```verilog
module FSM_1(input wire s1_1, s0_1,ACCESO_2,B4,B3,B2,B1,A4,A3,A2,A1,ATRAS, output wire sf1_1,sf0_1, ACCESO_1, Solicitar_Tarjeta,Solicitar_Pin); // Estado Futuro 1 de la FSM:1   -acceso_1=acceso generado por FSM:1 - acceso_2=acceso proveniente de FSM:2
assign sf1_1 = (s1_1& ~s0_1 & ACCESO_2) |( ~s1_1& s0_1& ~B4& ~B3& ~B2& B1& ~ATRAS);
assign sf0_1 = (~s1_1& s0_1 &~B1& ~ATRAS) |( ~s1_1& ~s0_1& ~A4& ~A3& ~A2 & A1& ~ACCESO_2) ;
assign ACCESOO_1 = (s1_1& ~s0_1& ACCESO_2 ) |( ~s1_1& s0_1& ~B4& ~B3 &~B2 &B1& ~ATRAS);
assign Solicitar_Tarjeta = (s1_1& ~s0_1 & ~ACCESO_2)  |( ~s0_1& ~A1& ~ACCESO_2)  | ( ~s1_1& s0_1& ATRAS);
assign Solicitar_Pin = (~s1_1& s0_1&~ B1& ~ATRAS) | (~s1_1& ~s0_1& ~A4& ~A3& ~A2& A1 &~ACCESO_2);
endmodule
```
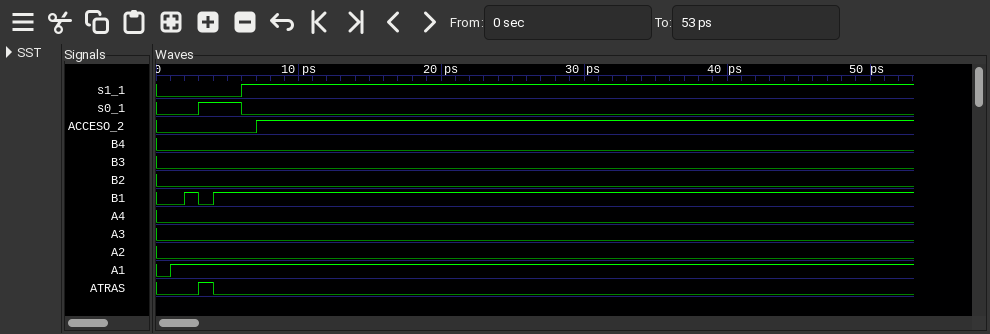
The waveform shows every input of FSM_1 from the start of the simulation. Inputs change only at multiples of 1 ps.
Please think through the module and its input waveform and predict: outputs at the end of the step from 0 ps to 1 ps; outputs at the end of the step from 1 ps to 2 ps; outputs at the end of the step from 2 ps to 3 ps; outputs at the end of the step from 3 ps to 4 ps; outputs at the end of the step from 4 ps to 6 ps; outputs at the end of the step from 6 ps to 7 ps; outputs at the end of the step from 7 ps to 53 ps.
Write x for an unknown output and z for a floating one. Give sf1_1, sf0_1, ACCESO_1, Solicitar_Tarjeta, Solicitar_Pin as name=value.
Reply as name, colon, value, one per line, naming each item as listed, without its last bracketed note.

outputs at the end of the step from 0 ps to 1 ps: sf1_1=0, sf0_1=0, ACCESO_1=z, Solicitar_Tarjeta=1, Solicitar_Pin=0
outputs at the end of the step from 1 ps to 2 ps: sf1_1=0, sf0_1=1, ACCESO_1=z, Solicitar_Tarjeta=0, Solicitar_Pin=1
outputs at the end of the step from 2 ps to 3 ps: sf1_1=0, sf0_1=1, ACCESO_1=z, Solicitar_Tarjeta=0, Solicitar_Pin=1
outputs at the end of the step from 3 ps to 4 ps: sf1_1=0, sf0_1=0, ACCESO_1=z, Solicitar_Tarjeta=1, Solicitar_Pin=0
outputs at the end of the step from 4 ps to 6 ps: sf1_1=1, sf0_1=0, ACCESO_1=z, Solicitar_Tarjeta=0, Solicitar_Pin=0
outputs at the end of the step from 6 ps to 7 ps: sf1_1=0, sf0_1=0, ACCESO_1=z, Solicitar_Tarjeta=1, Solicitar_Pin=0
outputs at the end of the step from 7 ps to 53 ps: sf1_1=1, sf0_1=0, ACCESO_1=z, Solicitar_Tarjeta=0, Solicitar_Pin=0
